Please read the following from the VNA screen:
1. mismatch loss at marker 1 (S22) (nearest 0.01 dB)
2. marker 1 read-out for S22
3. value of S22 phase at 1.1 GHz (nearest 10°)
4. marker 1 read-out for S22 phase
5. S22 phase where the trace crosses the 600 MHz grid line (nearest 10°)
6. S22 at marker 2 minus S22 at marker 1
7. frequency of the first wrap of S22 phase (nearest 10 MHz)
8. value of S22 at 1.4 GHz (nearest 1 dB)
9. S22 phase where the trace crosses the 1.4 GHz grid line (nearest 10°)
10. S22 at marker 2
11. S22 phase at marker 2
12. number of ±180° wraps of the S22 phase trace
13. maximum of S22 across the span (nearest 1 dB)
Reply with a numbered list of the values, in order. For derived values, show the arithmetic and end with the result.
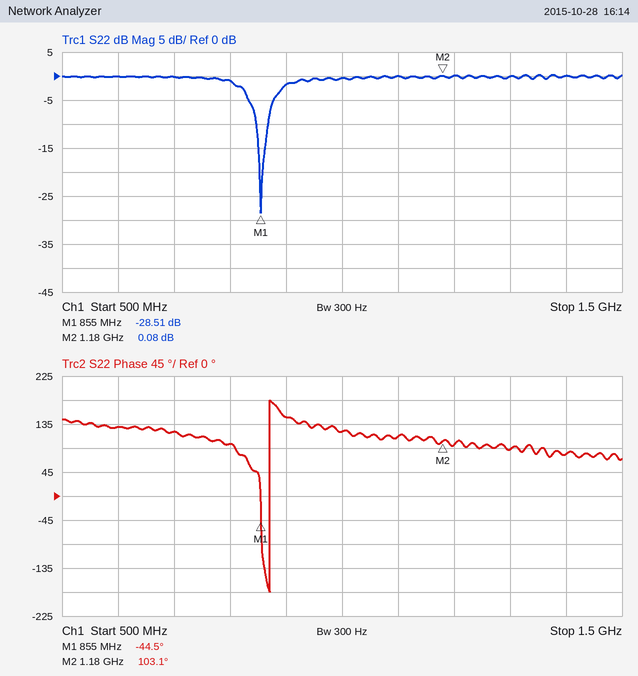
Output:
1. −10 log10(1 − 10^(-28.51/10)) ≈ 0.01 dB
2. -28.51 dB
3. 110°
4. -44.5°
5. 130°
6. 0.08 − (-28.51) = 28.59 dB
7. 870 MHz
8. 0 dB
9. 80°
10. 0.08 dB
11. 103.1°
12. 1
13. 0 dB
